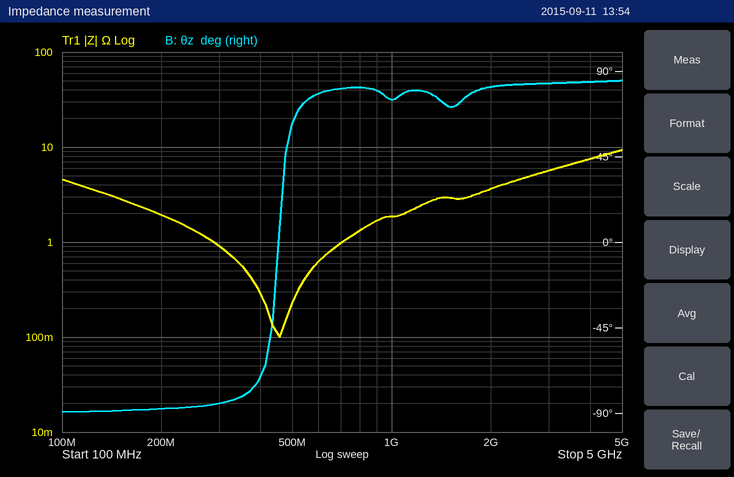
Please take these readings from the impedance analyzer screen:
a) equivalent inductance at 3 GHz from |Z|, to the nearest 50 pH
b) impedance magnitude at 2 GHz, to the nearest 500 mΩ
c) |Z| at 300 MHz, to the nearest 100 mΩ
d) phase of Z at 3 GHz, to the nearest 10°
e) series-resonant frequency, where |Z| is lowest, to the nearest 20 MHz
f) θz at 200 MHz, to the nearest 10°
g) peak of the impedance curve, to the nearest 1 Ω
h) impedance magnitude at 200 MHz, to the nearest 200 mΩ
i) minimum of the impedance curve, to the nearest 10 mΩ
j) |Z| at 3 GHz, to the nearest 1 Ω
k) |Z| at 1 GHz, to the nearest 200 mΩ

300 pH
3.5 Ω
900 mΩ
80°
460 MHz
-90°
9 Ω
2.0 Ω
100 mΩ
6 Ω
1.8 Ω
